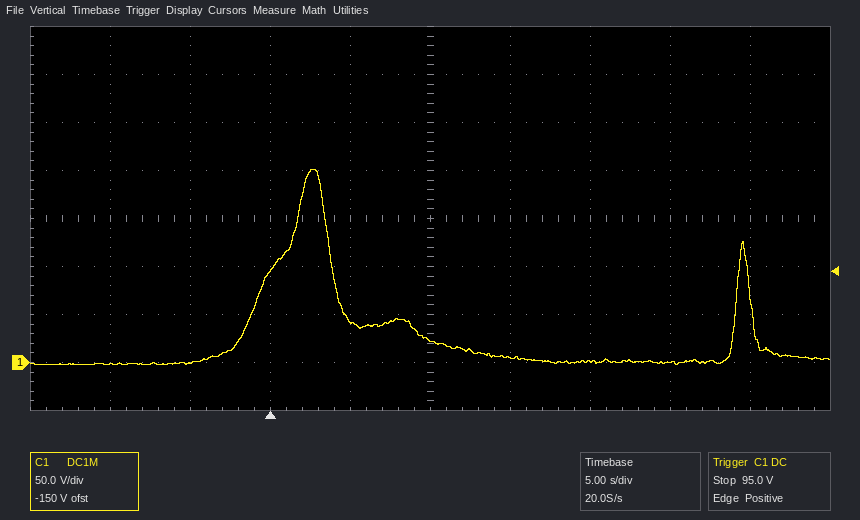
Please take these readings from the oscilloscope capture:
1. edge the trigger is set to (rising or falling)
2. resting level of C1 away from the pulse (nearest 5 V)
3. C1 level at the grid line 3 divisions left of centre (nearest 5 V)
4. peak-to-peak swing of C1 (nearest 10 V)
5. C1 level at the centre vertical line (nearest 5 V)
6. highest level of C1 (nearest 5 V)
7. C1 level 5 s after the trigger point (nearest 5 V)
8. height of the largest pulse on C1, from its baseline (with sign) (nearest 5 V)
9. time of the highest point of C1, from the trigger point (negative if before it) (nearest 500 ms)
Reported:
rising
0 V
0 V
200 V
25 V
200 V
45 V
+200 V
+2.5 s
